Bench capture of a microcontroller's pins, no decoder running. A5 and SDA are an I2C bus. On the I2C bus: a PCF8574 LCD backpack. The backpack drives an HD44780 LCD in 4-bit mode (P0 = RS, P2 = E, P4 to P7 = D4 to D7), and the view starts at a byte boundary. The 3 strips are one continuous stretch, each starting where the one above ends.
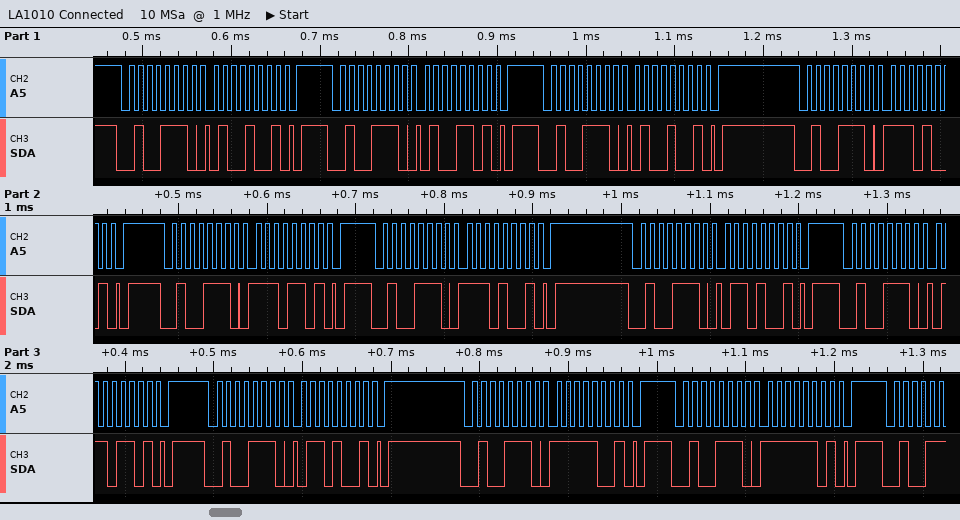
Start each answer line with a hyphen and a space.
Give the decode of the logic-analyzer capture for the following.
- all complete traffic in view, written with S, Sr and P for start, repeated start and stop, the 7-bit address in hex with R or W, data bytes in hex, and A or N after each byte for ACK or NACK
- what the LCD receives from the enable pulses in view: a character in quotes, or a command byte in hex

- S 27W A 49 A P S 27W A 4D A P S 27W A 49 A P S 27W A E9 A P S 27W A ED A P S 27W A E9 A P S 27W A 69 A P S 27W A 6D A P S 27W A 69 A P S 27W A F9 A P S 27W A FD A P
- 'N'
